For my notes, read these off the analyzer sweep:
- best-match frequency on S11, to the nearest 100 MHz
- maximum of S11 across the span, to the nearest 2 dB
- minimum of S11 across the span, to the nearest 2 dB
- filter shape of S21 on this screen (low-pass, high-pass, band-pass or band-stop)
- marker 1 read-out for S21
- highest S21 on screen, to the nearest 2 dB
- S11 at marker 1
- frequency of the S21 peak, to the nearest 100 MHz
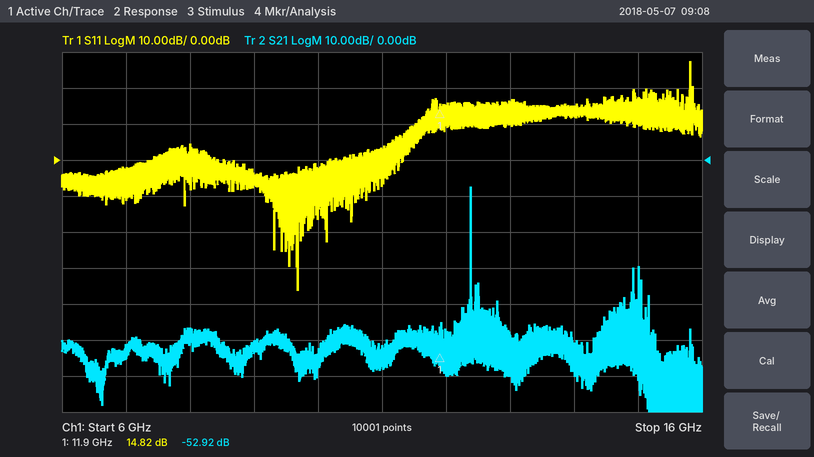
9.7 GHz
28 dB
-36 dB
band-pass
-52.92 dB
-8 dB
14.82 dB
12.4 GHz
